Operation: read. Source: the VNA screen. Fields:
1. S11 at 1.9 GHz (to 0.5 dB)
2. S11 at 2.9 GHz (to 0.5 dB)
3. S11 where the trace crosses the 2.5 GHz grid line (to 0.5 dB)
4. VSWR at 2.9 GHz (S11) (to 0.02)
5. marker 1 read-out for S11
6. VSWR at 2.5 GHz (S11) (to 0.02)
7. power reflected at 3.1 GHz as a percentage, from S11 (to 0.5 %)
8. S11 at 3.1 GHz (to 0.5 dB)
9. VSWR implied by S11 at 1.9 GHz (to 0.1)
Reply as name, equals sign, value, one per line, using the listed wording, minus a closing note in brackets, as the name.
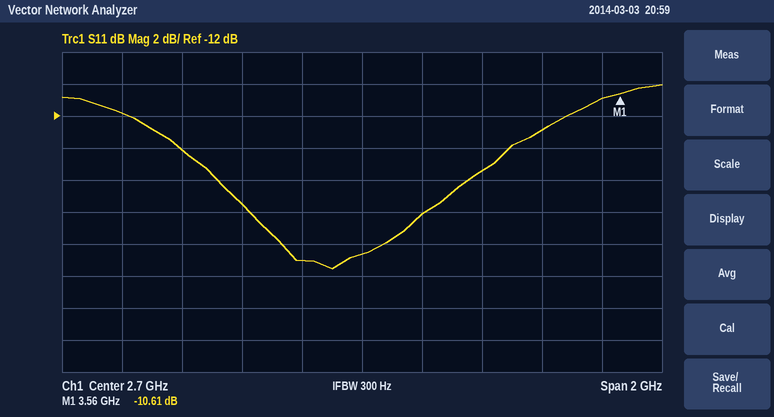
S11 at 1.9 GHz = -12.0 dB
S11 at 2.9 GHz = -18.0 dB
S11 where the trace crosses the 2.5 GHz grid line = -21.0 dB
VSWR at 2.9 GHz (S11) = 1.28
marker 1 read-out for S11 = -10.61 dB
VSWR at 2.5 GHz (S11) = 1.20
power reflected at 3.1 GHz as a percentage, from S11 = 3.0 %
S11 at 3.1 GHz = -15.5 dB
VSWR implied by S11 at 1.9 GHz = 1.7
